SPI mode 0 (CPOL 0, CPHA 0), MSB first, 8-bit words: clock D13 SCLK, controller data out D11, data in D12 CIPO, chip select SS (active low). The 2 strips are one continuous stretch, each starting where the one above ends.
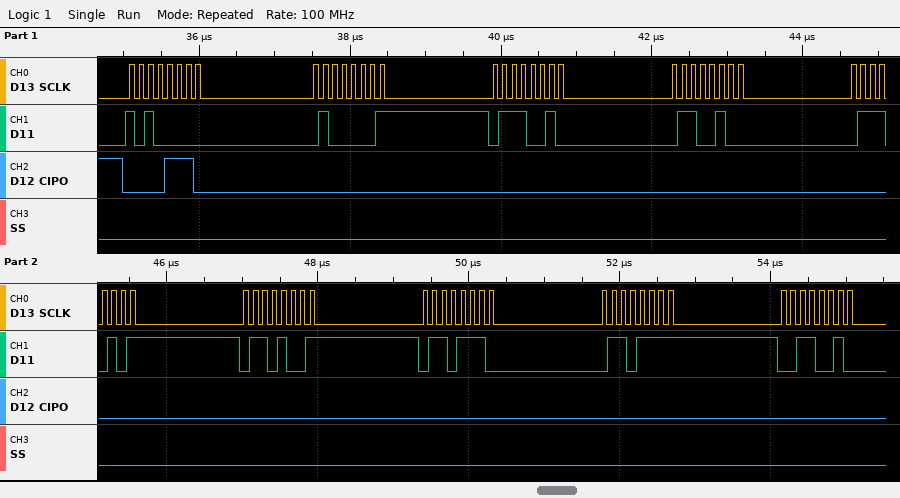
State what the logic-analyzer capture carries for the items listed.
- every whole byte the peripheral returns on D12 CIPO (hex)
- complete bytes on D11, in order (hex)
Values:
0E 00 00 00 00 00 00 00 00
A0 41 72 64 75 69 6E 6F 32
